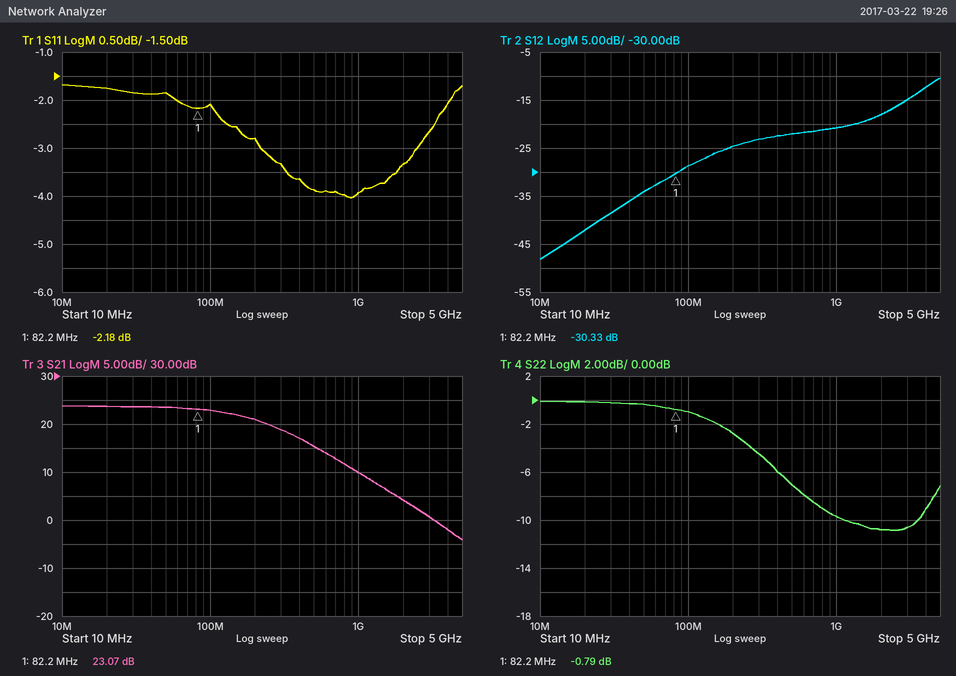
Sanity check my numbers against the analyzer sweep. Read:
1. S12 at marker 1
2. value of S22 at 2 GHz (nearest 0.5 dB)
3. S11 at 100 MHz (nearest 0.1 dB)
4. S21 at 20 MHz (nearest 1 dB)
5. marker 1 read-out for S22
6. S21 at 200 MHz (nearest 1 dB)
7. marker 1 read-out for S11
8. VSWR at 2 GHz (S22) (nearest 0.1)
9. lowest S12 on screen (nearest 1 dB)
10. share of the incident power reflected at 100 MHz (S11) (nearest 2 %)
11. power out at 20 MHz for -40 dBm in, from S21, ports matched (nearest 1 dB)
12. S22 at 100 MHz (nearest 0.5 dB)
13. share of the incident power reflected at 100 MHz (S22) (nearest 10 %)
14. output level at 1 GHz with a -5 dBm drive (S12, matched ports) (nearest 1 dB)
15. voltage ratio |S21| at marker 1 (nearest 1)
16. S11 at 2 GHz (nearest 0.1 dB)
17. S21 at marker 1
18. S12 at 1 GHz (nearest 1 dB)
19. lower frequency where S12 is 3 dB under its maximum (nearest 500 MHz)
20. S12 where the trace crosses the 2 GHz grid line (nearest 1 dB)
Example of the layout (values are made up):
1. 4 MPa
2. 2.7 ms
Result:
1. -30.33 dB
2. -11.0 dB
3. -2.1 dB
4. 24 dB
5. -0.79 dB
6. 21 dB
7. -2.18 dB
8. 1.8
9. -48 dB
10. 62 %
11. -16 dBm
12. -1.0 dB
13. 80 %
14. -26 dBm
15. 14
16. -3.3 dB
17. 23.07 dB
18. -21 dB
19. 3.5 GHz
20. -18 dB
